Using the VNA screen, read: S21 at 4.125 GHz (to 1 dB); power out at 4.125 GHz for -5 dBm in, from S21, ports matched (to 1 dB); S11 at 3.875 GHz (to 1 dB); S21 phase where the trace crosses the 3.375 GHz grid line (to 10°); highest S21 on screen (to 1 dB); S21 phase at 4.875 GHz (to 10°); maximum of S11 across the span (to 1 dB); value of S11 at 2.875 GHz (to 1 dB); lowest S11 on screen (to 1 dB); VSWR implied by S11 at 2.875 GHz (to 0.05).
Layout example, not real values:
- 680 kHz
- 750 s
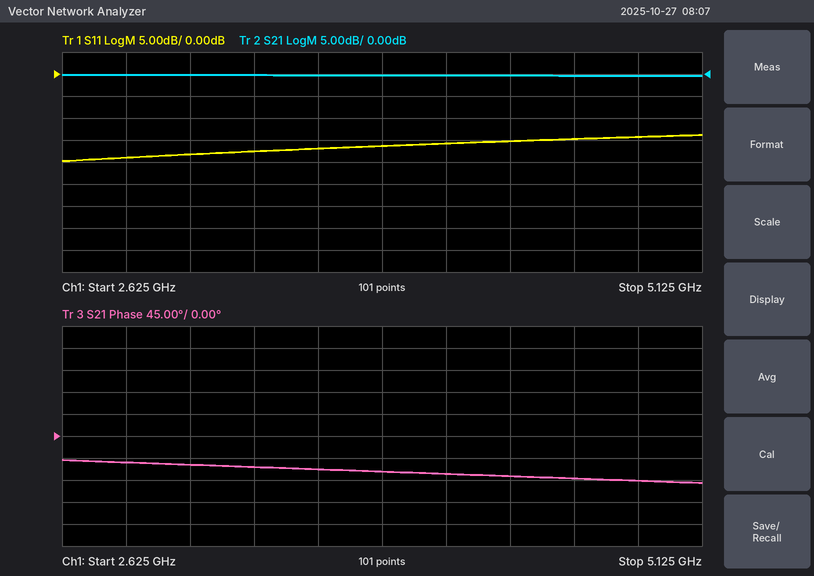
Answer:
- 0 dB
- -5 dBm
- -16 dB
- -60°
- 0 dB
- -90°
- -14 dB
- -19 dB
- -20 dB
- 1.25
